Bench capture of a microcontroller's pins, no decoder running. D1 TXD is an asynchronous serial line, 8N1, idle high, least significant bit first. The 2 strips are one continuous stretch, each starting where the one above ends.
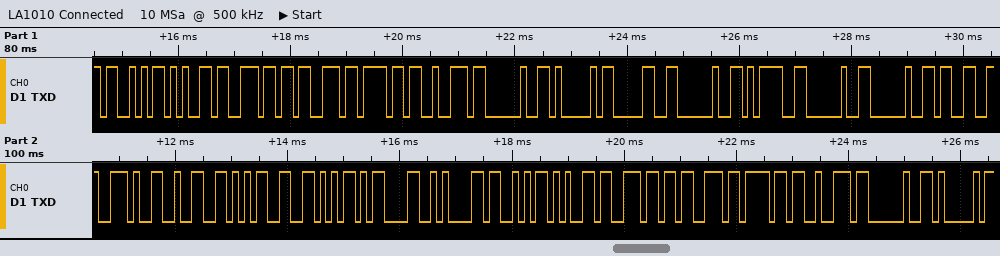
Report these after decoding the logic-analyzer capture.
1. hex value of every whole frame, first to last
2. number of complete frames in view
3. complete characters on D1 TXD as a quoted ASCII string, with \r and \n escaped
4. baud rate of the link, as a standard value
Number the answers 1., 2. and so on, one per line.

1. 53 65 6E 73 6F 72 20 41 30 20 3D 20 20 33 2E 32 35 56 0D 0A 53 65 6E 73 6F 72 20 41
2. 28
3. "Sensor A0 =  3.25V\r\nSensor A"
4. 9600 baud
